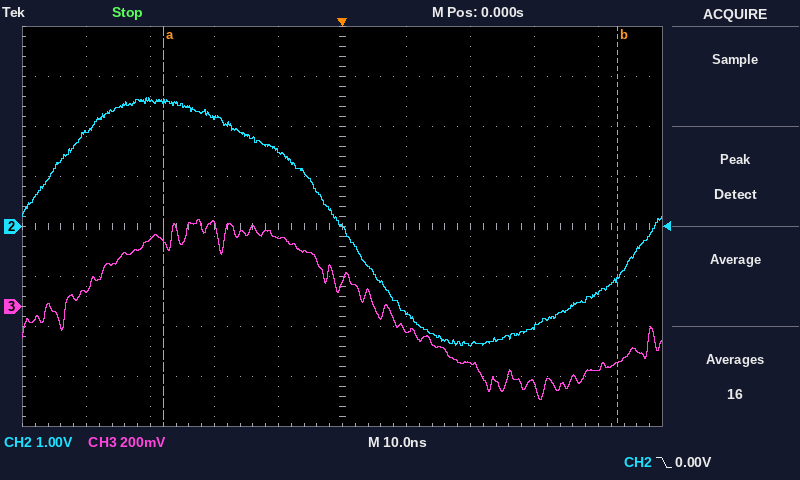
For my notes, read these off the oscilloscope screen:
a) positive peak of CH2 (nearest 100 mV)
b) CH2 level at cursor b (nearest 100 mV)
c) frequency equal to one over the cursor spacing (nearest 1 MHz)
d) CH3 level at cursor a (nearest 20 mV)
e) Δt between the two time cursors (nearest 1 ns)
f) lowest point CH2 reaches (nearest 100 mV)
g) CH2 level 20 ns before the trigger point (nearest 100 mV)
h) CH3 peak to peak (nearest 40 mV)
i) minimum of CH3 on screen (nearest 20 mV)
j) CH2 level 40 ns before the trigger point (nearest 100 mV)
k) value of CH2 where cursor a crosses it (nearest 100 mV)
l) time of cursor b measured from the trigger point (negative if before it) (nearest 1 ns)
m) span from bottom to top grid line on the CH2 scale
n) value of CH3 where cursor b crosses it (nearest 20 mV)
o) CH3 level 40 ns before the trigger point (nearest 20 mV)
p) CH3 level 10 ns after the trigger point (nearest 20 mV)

2.6 V
-1.0 V
14 MHz
260 mV
71 ns
-2.4 V
2.2 V
720 mV
-380 mV
1.9 V
2.5 V
+43 ns
8 V
-220 mV
60 mV
-100 mV
